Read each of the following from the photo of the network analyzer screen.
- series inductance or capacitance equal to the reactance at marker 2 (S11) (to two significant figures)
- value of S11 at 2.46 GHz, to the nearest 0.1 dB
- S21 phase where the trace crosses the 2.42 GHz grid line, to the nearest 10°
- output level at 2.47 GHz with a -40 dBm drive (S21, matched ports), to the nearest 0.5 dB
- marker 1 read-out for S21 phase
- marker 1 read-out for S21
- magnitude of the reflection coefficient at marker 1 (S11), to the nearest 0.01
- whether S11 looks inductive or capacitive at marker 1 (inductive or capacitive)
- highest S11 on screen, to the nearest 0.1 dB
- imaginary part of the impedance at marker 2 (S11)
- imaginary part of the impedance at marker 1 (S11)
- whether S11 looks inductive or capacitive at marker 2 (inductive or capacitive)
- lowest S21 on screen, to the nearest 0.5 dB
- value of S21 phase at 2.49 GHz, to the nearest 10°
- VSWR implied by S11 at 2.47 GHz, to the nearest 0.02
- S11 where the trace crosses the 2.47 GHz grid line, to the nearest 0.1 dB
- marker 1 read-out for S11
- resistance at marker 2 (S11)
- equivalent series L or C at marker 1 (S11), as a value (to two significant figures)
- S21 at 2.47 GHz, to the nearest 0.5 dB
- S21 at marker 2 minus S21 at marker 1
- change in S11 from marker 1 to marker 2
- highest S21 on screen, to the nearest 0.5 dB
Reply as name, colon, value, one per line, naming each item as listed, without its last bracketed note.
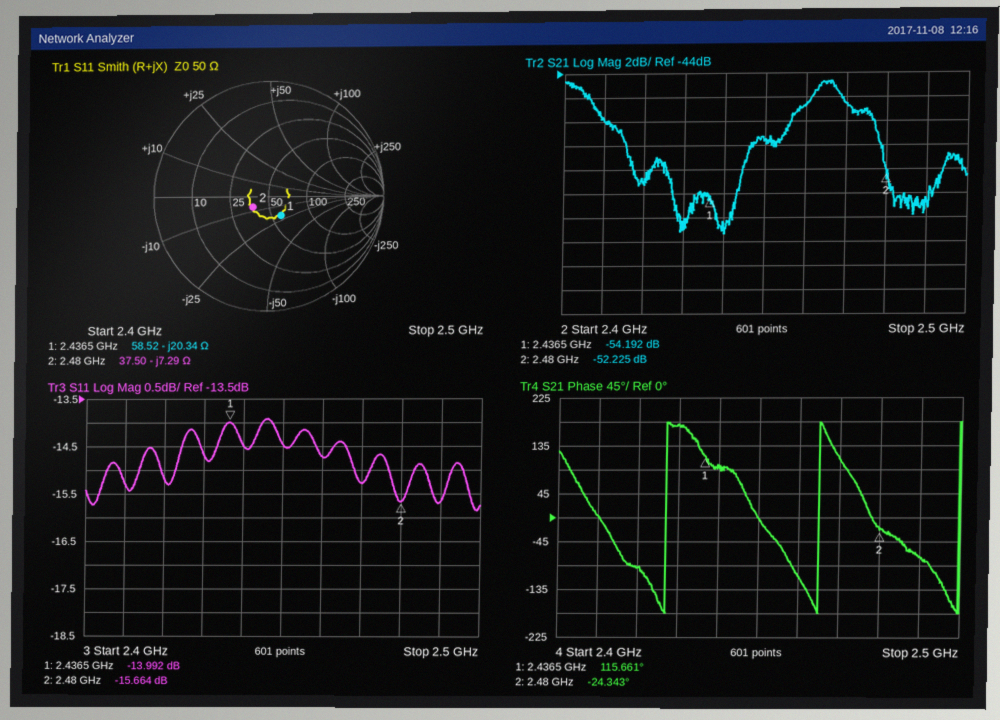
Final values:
series inductance or capacitance equal to the reactance at marker 2 (S11): 8.8 pF
value of S11 at 2.46 GHz, to the nearest 0.1 dB: -14.7 dB
S21 phase where the trace crosses the 2.42 GHz grid line, to the nearest 10°: -90°
output level at 2.47 GHz with a -40 dBm drive (S21, matched ports), to the nearest 0.5 dB: -86.5 dBm
marker 1 read-out for S21 phase: 115.661°
marker 1 read-out for S21: -54.192 dB
magnitude of the reflection coefficient at marker 1 (S11), to the nearest 0.01: 0.20
whether S11 looks inductive or capacitive at marker 1: capacitive
highest S11 on screen, to the nearest 0.1 dB: -13.9 dB
imaginary part of the impedance at marker 2: -7.29 Ω
imaginary part of the impedance at marker 1: -20.34 Ω
whether S11 looks inductive or capacitive at marker 2: capacitive
lowest S21 on screen, to the nearest 0.5 dB: -57.5 dB
value of S21 phase at 2.49 GHz, to the nearest 10°: -70°
VSWR implied by S11 at 2.47 GHz, to the nearest 0.02: 1.42
S11 where the trace crosses the 2.47 GHz grid line, to the nearest 0.1 dB: -15.3 dB
marker 1 read-out for S11: -13.992 dB
resistance at marker 2: 37.50 Ω
equivalent series L or C at marker 1 (S11), as a value: 3.2 pF
S21 at 2.47 GHz, to the nearest 0.5 dB: -46.5 dB
S21 at marker 2 minus S21 at marker 1: 1.967 dB
change in S11 from marker 1 to marker 2: -1.672 dB
highest S21 on screen, to the nearest 0.5 dB: -44.5 dB
